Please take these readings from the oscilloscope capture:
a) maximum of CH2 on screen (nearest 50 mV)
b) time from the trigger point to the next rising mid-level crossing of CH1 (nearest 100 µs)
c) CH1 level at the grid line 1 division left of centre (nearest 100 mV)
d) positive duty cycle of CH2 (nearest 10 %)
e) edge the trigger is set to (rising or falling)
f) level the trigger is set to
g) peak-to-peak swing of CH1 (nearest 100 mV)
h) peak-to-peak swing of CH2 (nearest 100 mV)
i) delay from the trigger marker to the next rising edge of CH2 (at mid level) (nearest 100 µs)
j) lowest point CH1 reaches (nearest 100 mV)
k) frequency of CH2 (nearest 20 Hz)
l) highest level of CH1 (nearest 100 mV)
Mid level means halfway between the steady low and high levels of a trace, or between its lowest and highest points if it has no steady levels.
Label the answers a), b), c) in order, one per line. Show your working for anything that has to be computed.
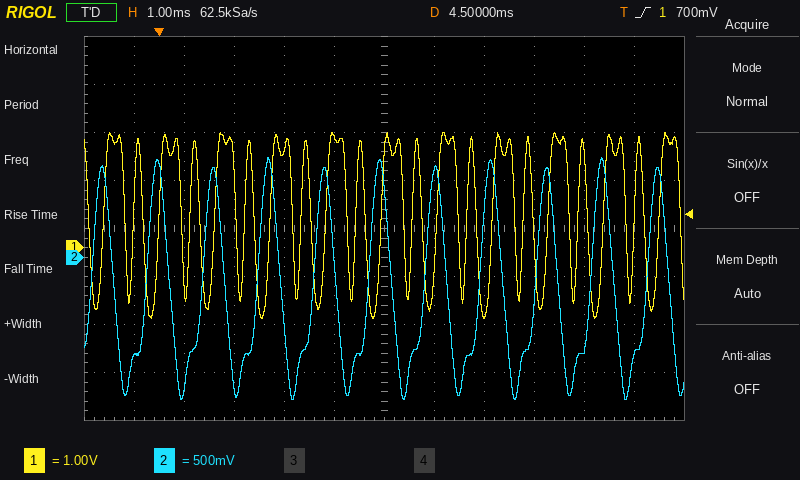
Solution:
a) 1.05 V
b) 600 µs
c) 2.3 V
d) 40 %
e) rising
f) 700 mV
g) 2.4 V − (-1.5 V) = 3.9 V
h) 2.50 V
i) 900 µs
j) -1.5 V
k) 900 Hz
l) 2.4 V
